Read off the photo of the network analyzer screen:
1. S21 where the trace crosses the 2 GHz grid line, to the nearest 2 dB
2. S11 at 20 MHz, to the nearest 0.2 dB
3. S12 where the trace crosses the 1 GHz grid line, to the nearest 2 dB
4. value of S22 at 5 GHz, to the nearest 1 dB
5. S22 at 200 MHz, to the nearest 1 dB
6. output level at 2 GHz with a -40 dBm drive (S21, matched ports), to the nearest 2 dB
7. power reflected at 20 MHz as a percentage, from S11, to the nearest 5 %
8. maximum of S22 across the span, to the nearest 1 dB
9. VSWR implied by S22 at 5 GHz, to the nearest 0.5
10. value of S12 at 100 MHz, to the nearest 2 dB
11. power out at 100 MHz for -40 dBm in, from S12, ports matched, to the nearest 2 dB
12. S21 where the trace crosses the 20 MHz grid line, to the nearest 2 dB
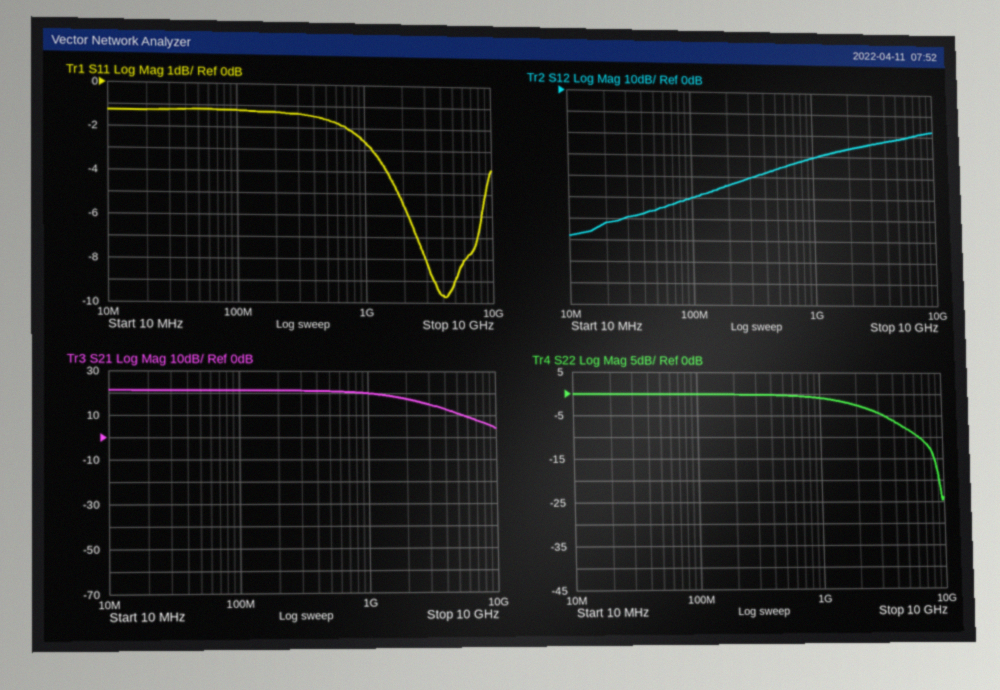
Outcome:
18 dB
-1.2 dB
-30 dB
-8 dB
0 dB
-22 dBm
75 %
0 dB
2.5
-50 dB
-90 dBm
22 dB
